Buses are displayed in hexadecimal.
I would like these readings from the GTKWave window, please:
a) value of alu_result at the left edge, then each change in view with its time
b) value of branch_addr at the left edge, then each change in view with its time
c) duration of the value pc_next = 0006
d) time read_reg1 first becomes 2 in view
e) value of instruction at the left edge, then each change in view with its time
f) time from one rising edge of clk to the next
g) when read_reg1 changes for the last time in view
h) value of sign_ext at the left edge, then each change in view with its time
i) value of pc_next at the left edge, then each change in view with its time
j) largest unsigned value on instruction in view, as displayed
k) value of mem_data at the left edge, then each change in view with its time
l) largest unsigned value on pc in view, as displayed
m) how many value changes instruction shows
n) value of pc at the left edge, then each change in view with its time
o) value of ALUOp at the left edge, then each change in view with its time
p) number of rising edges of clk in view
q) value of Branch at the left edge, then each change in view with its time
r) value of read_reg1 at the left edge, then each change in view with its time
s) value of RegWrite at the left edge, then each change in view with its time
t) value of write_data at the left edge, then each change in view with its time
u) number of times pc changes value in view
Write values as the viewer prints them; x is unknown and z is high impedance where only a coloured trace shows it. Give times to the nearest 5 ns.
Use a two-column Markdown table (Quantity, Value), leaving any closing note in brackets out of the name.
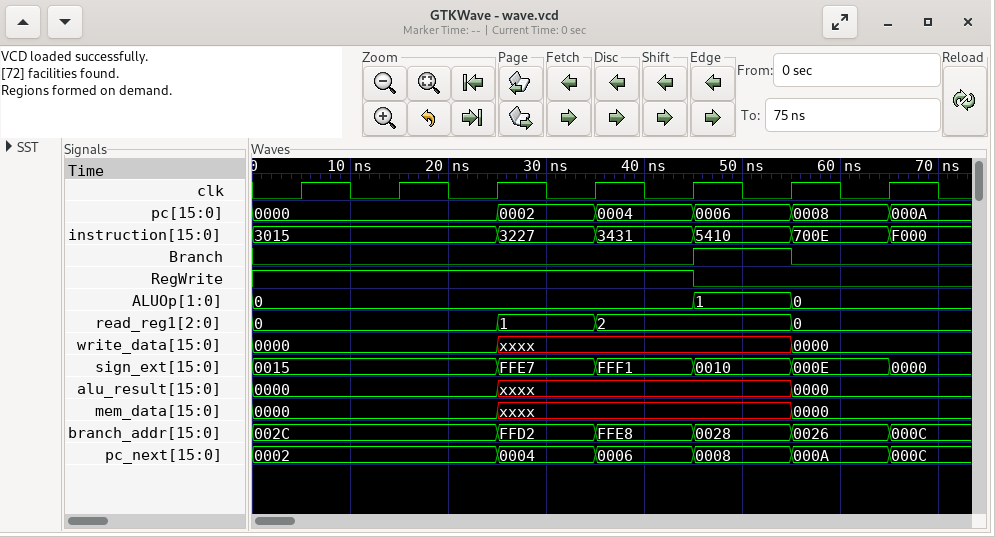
| Quantity | Value |
|---|---|
| value of alu_result at the left edge, then each change in view with its time | 0000, xxxx at 25 ns, 0000 at 55 ns |
| value of branch_addr at the left edge, then each change in view with its time | 002C, FFD2 at 25 ns, FFE8 at 35 ns, 0028 at 45 ns, 0026 at 55 ns, 000C at 65 ns |
| duration of the value pc_next = 0006 | 10 ns |
| time read_reg1 first becomes 2 in view | 35 ns |
| value of instruction at the left edge, then each change in view with its time | 3015, 3227 at 25 ns, 3431 at 35 ns, 5410 at 45 ns, 700E at 55 ns, F000 at 65 ns |
| time from one rising edge of clk to the next | 10 ns |
| when read_reg1 changes for the last time in view | 55 ns |
| value of sign_ext at the left edge, then each change in view with its time | 0015, FFE7 at 25 ns, FFF1 at 35 ns, 0010 at 45 ns, 000E at 55 ns, 0000 at 65 ns |
| value of pc_next at the left edge, then each change in view with its time | 0002, 0004 at 25 ns, 0006 at 35 ns, 0008 at 45 ns, 000A at 55 ns, 000C at 65 ns |
| largest unsigned value on instruction in view, as displayed | F000 |
| value of mem_data at the left edge, then each change in view with its time | 0000, xxxx at 25 ns, 0000 at 55 ns |
| largest unsigned value on pc in view, as displayed | 000A |
| how many value changes instruction shows | 5 |
| value of pc at the left edge, then each change in view with its time | 0000, 0002 at 25 ns, 0004 at 35 ns, 0006 at 45 ns, 0008 at 55 ns, 000A at 65 ns |
| value of ALUOp at the left edge, then each change in view with its time | 0, 1 at 45 ns, 0 at 55 ns |
| number of rising edges of clk in view | 7 |
| value of Branch at the left edge, then each change in view with its time | 0, 1 at 45 ns, 0 at 55 ns |
| value of read_reg1 at the left edge, then each change in view with its time | 0, 1 at 25 ns, 2 at 35 ns, 0 at 55 ns |
| value of RegWrite at the left edge, then each change in view with its time | 1, 0 at 45 ns |
| value of write_data at the left edge, then each change in view with its time | 0000, xxxx at 25 ns, 0000 at 55 ns |
| number of times pc changes value in view | 5 |
